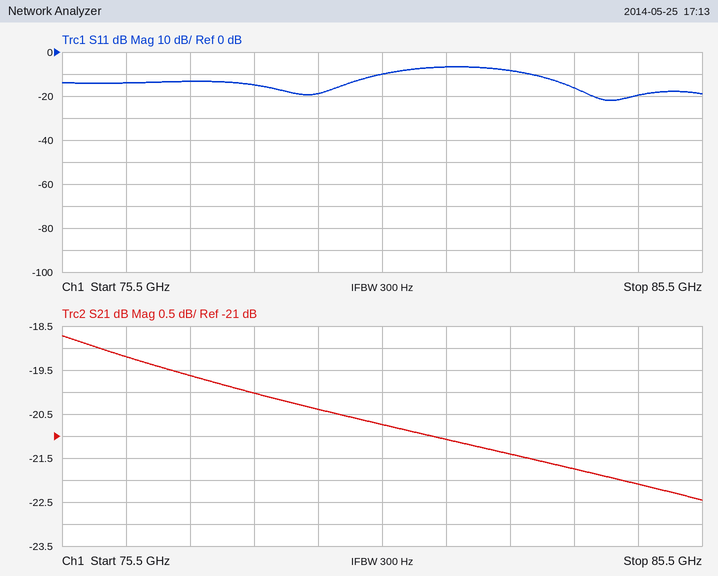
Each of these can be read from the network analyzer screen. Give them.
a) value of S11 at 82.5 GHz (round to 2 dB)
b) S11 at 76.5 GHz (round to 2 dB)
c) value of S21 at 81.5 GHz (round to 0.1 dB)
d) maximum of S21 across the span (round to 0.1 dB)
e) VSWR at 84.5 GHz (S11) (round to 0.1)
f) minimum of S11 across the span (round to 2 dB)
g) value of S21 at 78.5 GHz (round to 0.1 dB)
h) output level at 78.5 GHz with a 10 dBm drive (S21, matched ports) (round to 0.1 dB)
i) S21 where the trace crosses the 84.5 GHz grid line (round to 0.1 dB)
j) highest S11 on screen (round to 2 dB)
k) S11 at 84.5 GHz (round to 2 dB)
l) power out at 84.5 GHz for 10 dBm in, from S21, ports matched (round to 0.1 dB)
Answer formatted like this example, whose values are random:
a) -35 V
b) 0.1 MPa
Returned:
a) -8 dB
b) -14 dB
c) -21.1 dB
d) -18.7 dB
e) 1.2
f) -22 dB
g) -20.0 dB
h) -10.0 dBm
i) -22.1 dB
j) -6 dB
k) -20 dB
l) -12.1 dBm
